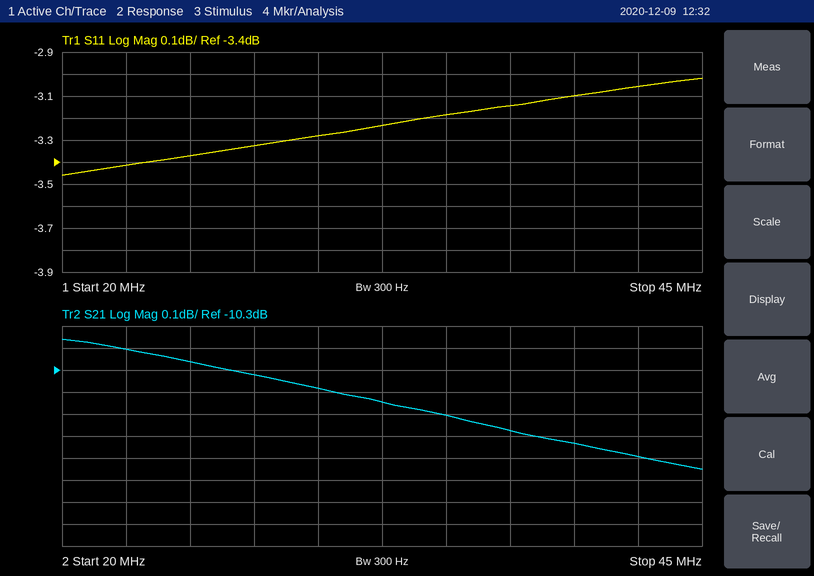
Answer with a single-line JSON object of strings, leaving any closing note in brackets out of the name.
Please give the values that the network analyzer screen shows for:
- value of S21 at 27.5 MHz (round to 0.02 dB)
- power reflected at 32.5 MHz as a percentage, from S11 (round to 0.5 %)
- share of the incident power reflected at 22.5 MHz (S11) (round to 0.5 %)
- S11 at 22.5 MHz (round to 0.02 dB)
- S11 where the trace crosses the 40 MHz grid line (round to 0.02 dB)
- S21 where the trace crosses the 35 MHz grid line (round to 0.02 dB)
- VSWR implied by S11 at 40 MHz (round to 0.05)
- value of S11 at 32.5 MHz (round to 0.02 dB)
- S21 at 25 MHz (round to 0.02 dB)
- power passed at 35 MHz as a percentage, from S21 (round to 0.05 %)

{"value of S21 at 27.5 MHz": "-10.32 dB", "power reflected at 32.5 MHz as a percentage, from S11": "47.5 %", "share of the incident power reflected at 22.5 MHz (S11)": "45.5 %", "S11 at 22.5 MHz": "-3.42 dB", "S11 where the trace crosses the 40 MHz grid line": "-3.10 dB", "S21 where the trace crosses the 35 MHz grid line": "-10.50 dB", "VSWR implied by S11 at 40 MHz": "5.65", "value of S11 at 32.5 MHz": "-3.24 dB", "S21 at 25 MHz": "-10.26 dB", "power passed at 35 MHz as a percentage, from S21": "8.90 %"}
